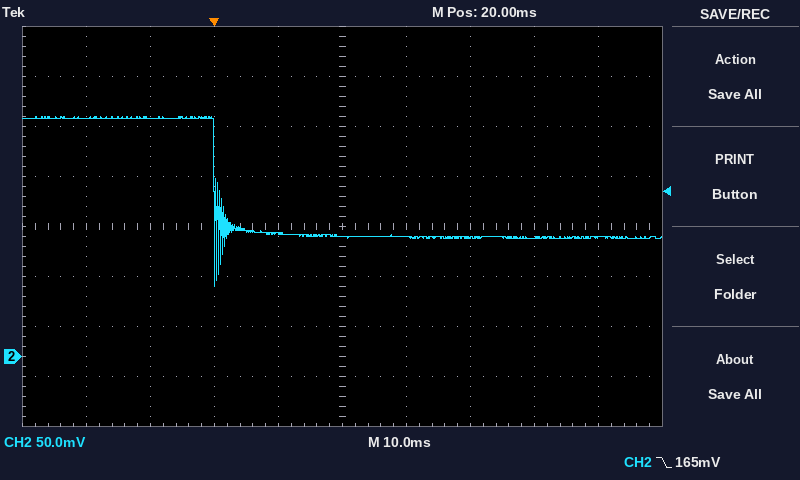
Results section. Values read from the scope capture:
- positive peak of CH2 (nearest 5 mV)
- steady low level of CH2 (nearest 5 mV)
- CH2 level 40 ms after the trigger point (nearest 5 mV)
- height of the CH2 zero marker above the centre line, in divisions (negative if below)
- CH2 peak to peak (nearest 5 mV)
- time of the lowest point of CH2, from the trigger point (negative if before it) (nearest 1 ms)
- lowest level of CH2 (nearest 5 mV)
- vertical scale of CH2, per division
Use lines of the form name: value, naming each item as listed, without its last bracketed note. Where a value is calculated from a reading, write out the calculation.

positive peak of CH2: 240 mV
steady low level of CH2: 120 mV
CH2 level 40 ms after the trigger point: 120 mV
height of the CH2 zero marker above the centre line, in divisions: -2.6 div
CH2 peak to peak: 240 mV − (70 mV) = 170 mV
time of the lowest point of CH2, from the trigger point (negative if before it): 0 ms
lowest level of CH2: 70 mV
vertical scale of CH2, per division: 50 mV
